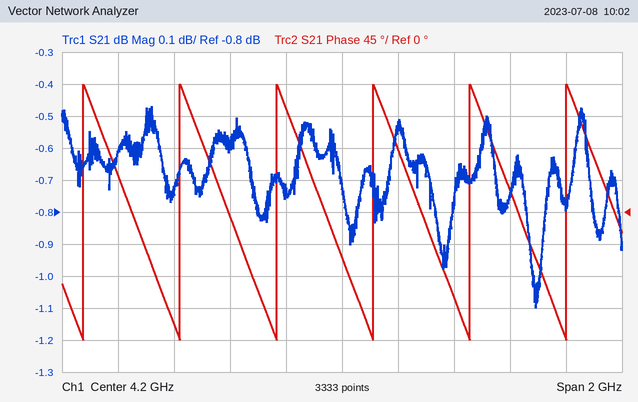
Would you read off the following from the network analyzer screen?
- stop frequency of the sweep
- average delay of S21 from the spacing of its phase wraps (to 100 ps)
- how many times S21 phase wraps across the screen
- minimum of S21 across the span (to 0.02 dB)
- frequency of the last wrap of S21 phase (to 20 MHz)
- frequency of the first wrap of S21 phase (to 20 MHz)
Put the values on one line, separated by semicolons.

5.2 GHz; 2.9 ns; 6; -1.10 dB; 5.00 GHz; 3.28 GHz
